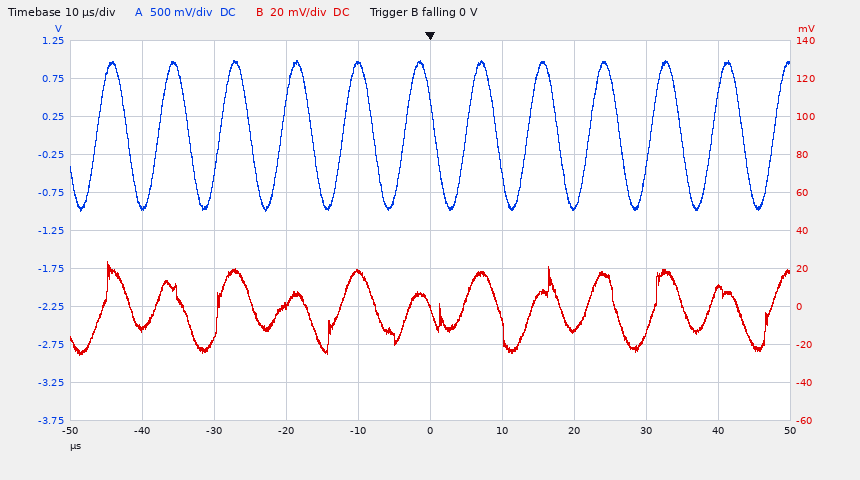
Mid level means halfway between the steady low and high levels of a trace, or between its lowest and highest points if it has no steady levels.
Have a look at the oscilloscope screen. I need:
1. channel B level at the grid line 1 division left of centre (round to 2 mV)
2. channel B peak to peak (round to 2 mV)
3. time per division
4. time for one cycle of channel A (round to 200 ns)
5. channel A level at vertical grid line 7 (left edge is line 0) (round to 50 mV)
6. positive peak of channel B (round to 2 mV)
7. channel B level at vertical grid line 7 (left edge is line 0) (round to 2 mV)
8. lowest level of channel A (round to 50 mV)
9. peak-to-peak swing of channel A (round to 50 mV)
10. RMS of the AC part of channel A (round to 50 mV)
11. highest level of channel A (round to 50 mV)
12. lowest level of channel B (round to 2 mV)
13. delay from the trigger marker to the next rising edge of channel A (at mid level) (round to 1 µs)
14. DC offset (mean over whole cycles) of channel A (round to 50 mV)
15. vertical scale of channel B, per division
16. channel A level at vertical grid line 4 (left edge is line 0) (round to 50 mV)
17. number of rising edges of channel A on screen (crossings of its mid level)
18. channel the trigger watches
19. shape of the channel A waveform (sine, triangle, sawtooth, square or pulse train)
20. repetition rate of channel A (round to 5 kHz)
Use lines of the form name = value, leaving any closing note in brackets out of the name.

channel B level at the grid line 1 division left of centre = 18 mV
channel B peak to peak = 50 mV
time per division = 10 µs
time for one cycle of channel A = 8.6 µs
channel A level at vertical grid line 7 (left edge is line 0) = -950 mV
positive peak of channel B = 24 mV
channel B level at vertical grid line 7 (left edge is line 0) = -12 mV
lowest level of channel A = -1.00 V
peak-to-peak swing of channel A = 2.00 V
RMS of the AC part of channel A = 700 mV
highest level of channel A = 1.00 V
lowest level of channel B = -26 mV
delay from the trigger marker to the next rising edge of channel A (at mid level) = 5 µs
DC offset (mean over whole cycles) of channel A = 0 mV
vertical scale of channel B, per division = 20 mV
channel A level at vertical grid line 4 (left edge is line 0) = 950 mV
number of rising edges of channel A on screen = 12
channel the trigger watches = channel B
shape of the channel A waveform = sine
repetition rate of channel A = 115 kHz
